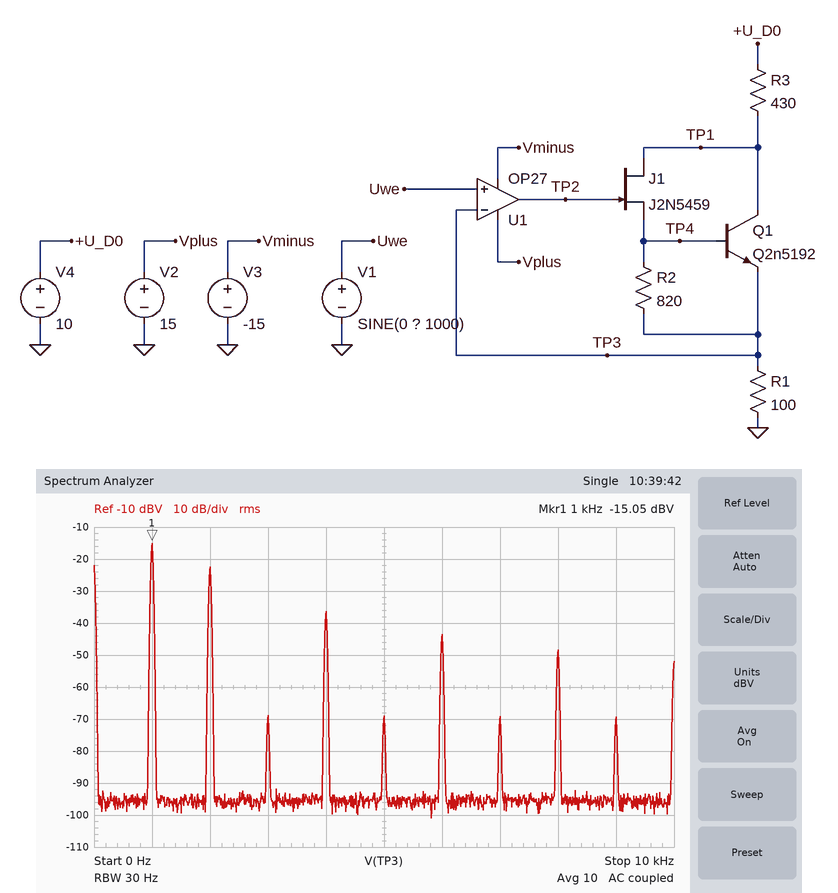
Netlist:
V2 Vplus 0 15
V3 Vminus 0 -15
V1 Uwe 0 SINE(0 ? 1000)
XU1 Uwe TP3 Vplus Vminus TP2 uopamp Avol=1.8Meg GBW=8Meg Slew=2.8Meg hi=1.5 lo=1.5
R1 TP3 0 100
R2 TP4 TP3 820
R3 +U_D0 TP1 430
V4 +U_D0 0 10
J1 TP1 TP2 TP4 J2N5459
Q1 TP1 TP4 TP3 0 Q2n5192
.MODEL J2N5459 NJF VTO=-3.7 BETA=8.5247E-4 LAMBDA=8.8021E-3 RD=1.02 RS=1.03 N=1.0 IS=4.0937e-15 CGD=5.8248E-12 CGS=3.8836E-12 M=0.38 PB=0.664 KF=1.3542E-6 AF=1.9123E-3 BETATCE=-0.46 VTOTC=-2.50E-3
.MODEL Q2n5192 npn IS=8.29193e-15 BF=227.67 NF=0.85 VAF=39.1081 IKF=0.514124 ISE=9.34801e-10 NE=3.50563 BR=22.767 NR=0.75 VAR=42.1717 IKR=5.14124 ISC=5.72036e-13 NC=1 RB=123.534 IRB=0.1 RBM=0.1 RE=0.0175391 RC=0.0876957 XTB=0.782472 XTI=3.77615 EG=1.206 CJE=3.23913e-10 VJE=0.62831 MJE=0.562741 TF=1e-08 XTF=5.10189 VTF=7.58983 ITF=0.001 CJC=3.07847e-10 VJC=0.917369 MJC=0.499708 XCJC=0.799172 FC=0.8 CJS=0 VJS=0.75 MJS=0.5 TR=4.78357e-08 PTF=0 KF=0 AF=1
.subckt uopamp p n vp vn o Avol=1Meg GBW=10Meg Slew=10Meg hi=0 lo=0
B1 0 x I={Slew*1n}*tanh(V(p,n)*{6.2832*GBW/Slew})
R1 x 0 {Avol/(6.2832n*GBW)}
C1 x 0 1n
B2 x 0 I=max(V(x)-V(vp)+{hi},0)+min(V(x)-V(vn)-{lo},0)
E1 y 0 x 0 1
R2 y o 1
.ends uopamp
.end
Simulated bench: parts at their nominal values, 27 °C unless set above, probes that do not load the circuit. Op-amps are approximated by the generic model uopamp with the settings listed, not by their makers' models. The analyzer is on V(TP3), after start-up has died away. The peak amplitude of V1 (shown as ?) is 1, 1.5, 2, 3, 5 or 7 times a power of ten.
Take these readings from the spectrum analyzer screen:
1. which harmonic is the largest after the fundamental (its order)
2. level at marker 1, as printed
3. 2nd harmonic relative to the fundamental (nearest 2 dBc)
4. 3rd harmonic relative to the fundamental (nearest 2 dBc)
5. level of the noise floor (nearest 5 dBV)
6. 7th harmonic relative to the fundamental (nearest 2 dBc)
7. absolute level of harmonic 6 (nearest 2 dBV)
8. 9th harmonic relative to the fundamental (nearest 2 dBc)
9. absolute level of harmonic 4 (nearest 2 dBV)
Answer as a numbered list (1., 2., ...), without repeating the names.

1. 2
2. -15.05 dBV
3. -8 dBc
4. -54 dBc
5. -95 dBV
6. -54 dBc
7. -44 dBV
8. -54 dBc
9. -36 dBV
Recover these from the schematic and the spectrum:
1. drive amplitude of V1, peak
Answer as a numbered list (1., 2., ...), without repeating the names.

1. 500 mV
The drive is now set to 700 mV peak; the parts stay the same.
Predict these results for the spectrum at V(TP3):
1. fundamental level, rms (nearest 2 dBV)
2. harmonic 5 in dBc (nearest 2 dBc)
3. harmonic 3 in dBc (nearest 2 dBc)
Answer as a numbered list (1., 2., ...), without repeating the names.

1. -12 dBV
2. -56 dBc
3. -56 dBc
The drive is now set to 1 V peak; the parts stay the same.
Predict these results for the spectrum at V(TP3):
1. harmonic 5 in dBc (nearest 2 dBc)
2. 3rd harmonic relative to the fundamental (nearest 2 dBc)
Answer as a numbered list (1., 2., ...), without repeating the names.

1. -60 dBc
2. -60 dBc
